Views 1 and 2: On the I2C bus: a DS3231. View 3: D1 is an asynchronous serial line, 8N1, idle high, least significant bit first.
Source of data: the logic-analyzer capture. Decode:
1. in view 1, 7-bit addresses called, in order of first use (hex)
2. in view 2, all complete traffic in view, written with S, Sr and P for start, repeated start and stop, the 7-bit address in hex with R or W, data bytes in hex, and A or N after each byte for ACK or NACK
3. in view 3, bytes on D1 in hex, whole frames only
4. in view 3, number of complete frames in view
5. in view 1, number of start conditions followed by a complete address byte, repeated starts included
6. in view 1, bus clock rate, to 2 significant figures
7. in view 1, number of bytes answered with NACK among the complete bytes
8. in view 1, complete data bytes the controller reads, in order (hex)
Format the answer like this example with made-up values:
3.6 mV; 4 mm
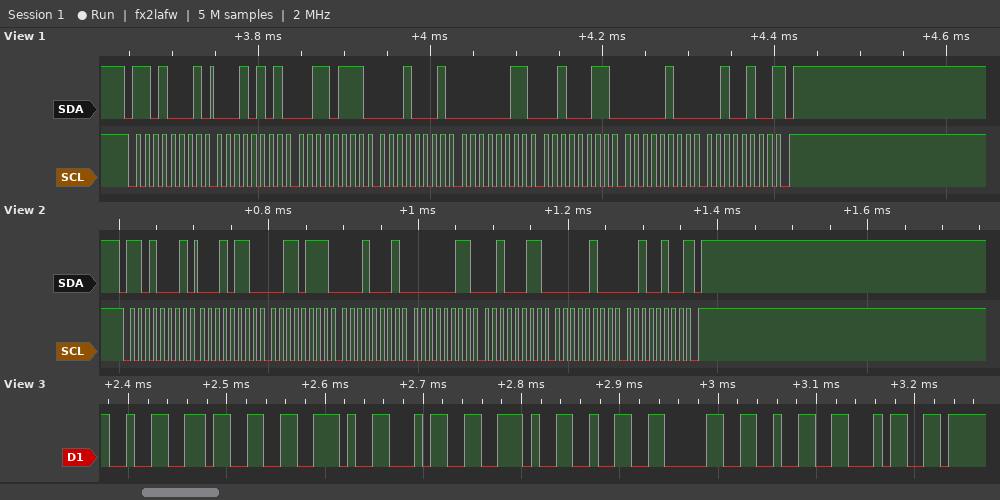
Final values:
0x68; S 68R A 16 A 37 A 11 A 03 A 23 A 04 A 24 N P; 32 33 2E 34 2E 32 30 32 34; 9; 1; 100 kHz; 1; 15 37 11 03 23 04 24
